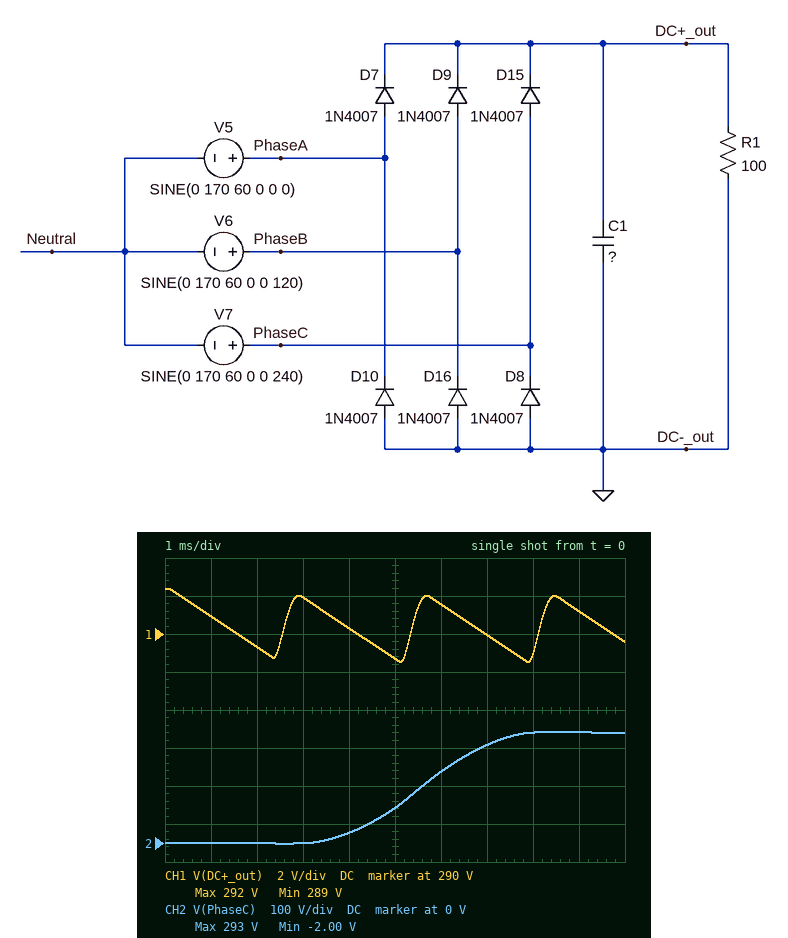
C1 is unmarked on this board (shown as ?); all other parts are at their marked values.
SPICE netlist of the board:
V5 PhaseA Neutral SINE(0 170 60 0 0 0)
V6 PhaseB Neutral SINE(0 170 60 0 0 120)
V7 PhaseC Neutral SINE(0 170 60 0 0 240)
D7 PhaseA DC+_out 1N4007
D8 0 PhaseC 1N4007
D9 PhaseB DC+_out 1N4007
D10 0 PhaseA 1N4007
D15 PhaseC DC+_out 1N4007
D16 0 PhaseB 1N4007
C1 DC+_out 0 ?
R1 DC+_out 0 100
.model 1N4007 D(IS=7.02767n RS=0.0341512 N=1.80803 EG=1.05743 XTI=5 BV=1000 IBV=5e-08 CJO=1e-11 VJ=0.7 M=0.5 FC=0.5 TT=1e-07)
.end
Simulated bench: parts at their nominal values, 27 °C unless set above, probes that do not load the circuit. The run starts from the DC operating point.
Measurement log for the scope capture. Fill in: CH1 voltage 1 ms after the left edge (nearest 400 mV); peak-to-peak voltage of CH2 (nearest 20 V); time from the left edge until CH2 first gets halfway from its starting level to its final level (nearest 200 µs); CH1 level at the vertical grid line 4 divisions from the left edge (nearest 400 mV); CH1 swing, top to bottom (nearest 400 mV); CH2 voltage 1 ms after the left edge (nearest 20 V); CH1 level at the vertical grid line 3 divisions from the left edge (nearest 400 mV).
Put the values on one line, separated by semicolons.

290.8 V; 300 V; 5.6 ms; 290.4 V; 4.0 V; 0 V; 292.0 V
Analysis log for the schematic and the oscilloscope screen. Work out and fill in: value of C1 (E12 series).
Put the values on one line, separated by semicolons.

1.8 mF
